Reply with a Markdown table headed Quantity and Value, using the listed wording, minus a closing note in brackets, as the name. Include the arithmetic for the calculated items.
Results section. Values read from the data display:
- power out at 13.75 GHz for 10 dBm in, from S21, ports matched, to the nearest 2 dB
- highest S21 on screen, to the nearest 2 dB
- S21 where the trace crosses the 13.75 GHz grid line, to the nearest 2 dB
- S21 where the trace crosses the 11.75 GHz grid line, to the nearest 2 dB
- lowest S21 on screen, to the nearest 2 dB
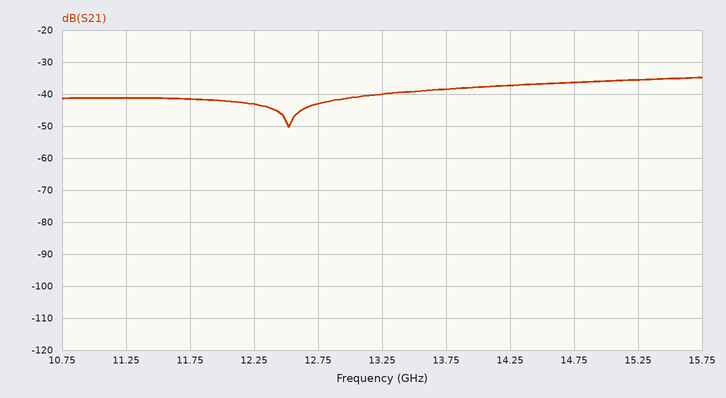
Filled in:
| Quantity | Value |
|---|---|
| power out at 13.75 GHz for 10 dBm in, from S21, ports matched, to the nearest 2 dB | 10 dBm + (-38 dB) = -28 dBm |
| highest S21 on screen, to the nearest 2 dB | -34 dB |
| S21 where the trace crosses the 13.75 GHz grid line, to the nearest 2 dB | -38 dB |
| S21 where the trace crosses the 11.75 GHz grid line, to the nearest 2 dB | -42 dB |
| lowest S21 on screen, to the nearest 2 dB | -50 dB |
